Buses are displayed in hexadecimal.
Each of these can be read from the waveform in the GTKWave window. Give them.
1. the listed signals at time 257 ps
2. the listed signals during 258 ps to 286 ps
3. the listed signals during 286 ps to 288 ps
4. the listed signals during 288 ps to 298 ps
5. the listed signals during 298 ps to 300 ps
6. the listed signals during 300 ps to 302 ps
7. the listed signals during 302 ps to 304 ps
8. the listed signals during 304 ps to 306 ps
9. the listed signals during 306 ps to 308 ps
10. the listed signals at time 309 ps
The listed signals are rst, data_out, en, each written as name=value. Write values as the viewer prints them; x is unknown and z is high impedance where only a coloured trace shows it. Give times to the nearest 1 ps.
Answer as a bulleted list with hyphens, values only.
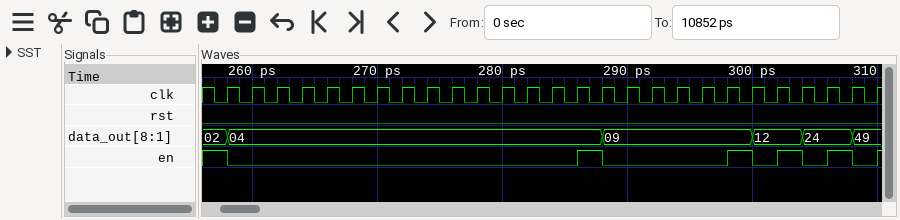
- rst=0, data_out=02, en=1
- rst=0, data_out=04, en=0
- rst=0, data_out=04, en=1
- rst=0, data_out=09, en=0
- rst=0, data_out=09, en=1
- rst=0, data_out=12, en=0
- rst=0, data_out=12, en=1
- rst=0, data_out=24, en=0
- rst=0, data_out=24, en=1
- rst=0, data_out=49, en=0
